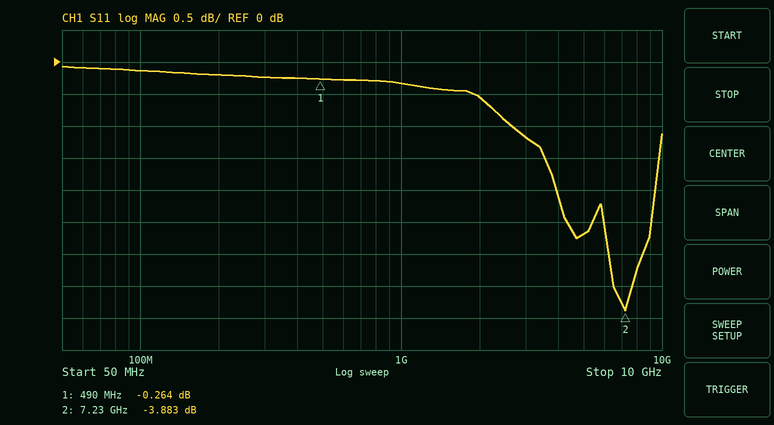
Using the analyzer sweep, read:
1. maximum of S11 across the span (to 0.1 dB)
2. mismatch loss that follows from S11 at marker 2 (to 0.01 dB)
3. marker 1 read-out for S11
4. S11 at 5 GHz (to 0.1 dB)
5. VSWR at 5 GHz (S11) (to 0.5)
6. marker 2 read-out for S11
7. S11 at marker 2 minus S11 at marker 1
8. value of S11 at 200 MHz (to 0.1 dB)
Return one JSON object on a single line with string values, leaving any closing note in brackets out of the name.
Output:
{"maximum of S11 across the span": "-0.1 dB", "mismatch loss that follows from S11 at marker 2": "2.28 dB", "marker 1 read-out for S11": "-0.264 dB", "S11 at 5 GHz": "-2.7 dB", "VSWR at 5 GHz (S11)": "6.5", "marker 2 read-out for S11": "-3.883 dB", "S11 at marker 2 minus S11 at marker 1": "-3.619 dB", "value of S11 at 200 MHz": "-0.2 dB"}
